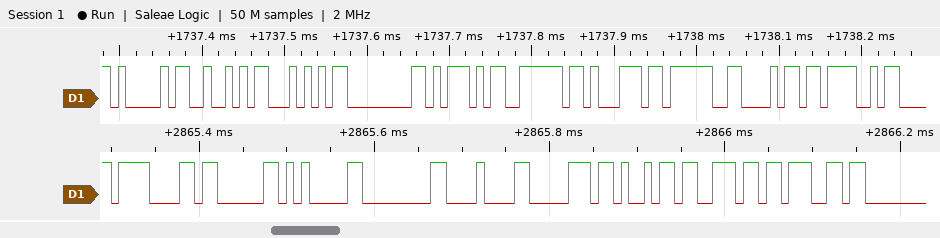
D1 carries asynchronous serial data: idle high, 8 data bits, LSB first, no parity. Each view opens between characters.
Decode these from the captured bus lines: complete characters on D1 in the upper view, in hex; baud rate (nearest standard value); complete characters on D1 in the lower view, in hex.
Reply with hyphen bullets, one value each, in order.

- 41, 52, 54, 00, 5D, 7E, 71, 3F, 68, 4F
- 115200 baud
- 0F, 03, 05, 00, 08, 70, 69, 6E, 67
